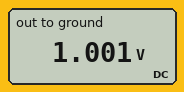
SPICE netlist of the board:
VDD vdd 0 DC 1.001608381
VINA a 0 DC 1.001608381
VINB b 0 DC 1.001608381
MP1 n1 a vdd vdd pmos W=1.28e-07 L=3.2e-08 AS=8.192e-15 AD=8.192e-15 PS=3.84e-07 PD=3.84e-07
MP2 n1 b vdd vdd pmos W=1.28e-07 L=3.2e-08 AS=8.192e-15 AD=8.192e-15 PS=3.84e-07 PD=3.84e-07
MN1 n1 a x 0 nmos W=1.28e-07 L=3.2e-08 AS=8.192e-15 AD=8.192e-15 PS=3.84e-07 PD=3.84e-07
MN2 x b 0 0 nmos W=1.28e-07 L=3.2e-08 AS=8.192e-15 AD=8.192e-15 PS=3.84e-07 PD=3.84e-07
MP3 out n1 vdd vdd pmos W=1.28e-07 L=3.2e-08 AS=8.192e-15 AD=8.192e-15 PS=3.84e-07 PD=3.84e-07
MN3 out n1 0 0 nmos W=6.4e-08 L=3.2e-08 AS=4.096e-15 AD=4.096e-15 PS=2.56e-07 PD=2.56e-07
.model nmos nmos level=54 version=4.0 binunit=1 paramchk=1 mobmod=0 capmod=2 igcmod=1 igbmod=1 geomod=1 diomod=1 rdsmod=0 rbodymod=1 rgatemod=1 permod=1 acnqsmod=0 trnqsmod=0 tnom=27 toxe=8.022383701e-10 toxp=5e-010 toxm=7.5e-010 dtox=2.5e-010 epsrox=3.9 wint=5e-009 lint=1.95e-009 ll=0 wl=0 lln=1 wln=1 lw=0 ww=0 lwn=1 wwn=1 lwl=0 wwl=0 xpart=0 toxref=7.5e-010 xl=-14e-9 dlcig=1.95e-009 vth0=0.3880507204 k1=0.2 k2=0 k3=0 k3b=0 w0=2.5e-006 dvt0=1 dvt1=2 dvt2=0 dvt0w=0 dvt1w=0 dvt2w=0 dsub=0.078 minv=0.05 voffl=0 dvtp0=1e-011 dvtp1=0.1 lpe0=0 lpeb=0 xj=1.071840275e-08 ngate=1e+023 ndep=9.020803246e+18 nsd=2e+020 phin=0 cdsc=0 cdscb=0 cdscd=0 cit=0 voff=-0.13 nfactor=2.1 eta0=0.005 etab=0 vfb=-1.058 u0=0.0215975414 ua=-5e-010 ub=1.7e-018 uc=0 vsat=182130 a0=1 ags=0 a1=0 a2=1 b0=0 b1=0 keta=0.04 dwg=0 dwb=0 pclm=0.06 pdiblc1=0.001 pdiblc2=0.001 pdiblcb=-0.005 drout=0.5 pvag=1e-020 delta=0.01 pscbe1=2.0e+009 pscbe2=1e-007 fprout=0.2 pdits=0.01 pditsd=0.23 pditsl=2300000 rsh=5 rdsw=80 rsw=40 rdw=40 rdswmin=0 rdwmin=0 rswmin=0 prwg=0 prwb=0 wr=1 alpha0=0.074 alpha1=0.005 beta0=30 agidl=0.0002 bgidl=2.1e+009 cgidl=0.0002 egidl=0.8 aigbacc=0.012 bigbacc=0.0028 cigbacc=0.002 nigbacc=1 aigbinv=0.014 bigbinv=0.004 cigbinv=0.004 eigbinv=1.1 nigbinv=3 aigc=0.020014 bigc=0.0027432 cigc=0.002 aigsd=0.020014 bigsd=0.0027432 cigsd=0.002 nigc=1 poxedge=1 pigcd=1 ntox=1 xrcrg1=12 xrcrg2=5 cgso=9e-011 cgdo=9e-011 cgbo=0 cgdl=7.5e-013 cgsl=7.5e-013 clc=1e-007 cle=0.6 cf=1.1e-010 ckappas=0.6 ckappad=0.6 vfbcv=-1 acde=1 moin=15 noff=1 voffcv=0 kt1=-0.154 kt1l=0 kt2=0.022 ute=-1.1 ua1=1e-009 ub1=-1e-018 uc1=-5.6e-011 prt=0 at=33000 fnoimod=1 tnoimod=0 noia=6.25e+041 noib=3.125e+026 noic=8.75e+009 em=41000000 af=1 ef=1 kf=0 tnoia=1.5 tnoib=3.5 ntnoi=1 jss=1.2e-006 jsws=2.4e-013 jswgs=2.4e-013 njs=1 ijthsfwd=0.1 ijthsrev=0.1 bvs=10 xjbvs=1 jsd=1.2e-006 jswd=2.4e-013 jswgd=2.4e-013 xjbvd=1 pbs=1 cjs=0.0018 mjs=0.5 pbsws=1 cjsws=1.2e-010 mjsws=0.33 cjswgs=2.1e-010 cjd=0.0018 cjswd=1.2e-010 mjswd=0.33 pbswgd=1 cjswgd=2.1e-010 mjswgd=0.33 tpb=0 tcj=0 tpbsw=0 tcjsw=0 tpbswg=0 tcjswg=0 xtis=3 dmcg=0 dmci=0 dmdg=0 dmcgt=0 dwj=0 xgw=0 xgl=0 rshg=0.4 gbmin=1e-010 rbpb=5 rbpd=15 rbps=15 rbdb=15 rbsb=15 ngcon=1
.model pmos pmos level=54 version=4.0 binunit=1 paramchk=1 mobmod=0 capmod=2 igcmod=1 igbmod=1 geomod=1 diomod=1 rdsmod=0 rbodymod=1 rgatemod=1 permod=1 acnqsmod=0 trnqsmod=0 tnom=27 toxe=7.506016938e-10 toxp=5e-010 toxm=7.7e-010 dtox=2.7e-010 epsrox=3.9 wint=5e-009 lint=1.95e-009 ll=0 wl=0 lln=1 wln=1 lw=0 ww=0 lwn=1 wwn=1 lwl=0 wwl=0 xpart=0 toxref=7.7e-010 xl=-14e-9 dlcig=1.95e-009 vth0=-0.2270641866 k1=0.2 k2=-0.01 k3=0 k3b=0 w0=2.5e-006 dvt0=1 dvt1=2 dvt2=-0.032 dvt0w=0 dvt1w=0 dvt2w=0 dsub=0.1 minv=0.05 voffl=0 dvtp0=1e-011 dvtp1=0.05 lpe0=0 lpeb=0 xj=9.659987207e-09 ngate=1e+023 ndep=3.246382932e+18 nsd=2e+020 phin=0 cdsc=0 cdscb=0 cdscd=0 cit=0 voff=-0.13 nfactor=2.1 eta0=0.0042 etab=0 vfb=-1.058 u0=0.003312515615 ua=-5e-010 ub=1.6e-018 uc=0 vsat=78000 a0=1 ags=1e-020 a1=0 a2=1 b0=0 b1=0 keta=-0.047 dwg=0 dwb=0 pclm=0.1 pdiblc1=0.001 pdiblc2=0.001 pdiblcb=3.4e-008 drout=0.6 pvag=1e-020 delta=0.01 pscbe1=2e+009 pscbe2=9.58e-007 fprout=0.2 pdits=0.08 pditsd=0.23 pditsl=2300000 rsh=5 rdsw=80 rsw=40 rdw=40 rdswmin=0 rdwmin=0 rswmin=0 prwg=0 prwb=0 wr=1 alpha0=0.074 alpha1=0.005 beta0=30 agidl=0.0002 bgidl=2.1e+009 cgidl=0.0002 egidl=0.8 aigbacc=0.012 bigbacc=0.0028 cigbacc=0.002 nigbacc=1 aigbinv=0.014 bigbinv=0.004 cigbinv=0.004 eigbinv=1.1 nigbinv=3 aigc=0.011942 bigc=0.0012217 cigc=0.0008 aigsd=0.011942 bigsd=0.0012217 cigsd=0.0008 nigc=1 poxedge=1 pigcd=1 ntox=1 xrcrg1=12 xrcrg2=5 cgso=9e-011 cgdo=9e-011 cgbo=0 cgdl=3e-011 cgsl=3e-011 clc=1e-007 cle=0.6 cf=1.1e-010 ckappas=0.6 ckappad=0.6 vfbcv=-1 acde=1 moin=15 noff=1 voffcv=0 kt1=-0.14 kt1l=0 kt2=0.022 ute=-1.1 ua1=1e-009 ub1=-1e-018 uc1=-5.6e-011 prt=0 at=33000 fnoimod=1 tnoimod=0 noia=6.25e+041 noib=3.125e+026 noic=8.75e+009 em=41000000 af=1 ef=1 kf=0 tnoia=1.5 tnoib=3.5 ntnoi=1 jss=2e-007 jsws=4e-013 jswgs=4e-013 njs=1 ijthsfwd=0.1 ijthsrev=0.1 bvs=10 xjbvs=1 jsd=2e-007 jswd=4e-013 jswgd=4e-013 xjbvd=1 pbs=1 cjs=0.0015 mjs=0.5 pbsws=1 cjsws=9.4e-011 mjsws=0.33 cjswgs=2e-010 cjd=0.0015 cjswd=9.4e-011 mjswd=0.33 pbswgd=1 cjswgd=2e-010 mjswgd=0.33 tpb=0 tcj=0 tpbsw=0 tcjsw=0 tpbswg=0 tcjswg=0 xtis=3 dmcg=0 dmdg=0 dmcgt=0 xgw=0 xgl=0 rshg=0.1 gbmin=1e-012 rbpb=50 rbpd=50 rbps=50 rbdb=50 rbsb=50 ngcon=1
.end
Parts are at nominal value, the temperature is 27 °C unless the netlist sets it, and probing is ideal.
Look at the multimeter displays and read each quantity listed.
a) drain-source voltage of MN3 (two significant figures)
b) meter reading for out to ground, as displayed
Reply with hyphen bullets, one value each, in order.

- 1.0 V
- 1.001 V
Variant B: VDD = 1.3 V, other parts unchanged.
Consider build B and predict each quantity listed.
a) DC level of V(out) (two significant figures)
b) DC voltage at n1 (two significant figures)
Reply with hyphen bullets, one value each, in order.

- 1.3 V
- 150 mV
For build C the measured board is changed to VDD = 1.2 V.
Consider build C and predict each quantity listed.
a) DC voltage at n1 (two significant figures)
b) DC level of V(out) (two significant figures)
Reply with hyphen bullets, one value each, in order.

- 52 mV
- 1.2 V
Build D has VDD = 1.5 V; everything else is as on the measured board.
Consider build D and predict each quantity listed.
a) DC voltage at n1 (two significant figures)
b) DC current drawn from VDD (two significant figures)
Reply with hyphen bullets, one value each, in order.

- 430 mV
- 140 µA
